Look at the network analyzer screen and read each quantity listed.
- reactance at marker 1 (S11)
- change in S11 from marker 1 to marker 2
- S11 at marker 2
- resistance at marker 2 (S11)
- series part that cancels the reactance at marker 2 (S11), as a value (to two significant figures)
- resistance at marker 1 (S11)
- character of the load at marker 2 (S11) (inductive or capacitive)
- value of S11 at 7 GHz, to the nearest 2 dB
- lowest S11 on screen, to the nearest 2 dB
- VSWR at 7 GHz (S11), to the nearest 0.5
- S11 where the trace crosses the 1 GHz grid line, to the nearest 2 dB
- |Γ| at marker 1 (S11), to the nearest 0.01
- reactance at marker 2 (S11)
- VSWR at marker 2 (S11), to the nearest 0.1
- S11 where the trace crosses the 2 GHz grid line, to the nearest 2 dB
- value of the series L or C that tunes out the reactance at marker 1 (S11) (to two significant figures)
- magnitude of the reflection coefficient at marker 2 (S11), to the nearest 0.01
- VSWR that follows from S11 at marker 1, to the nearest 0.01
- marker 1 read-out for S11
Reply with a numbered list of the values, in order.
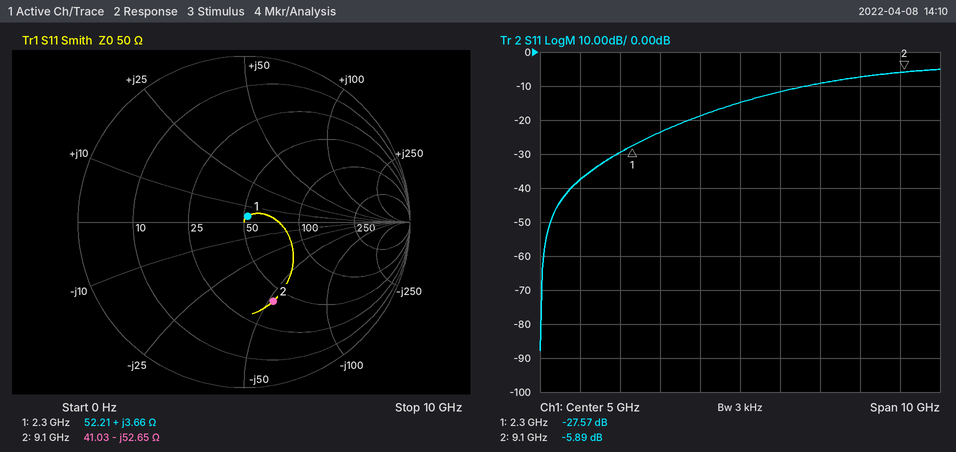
1. +3.66 Ω
2. 21.68 dB
3. -5.89 dB
4. 41.03 Ω
5. 920 pH
6. 52.21 Ω
7. capacitive
8. -10 dB
9. -88 dB
10. 2.0
11. -38 dB
12. 0.04
13. -52.65 Ω
14. 3.1
15. -30 dB
16. 19 pF
17. 0.51
18. 1.09
19. -27.57 dB
